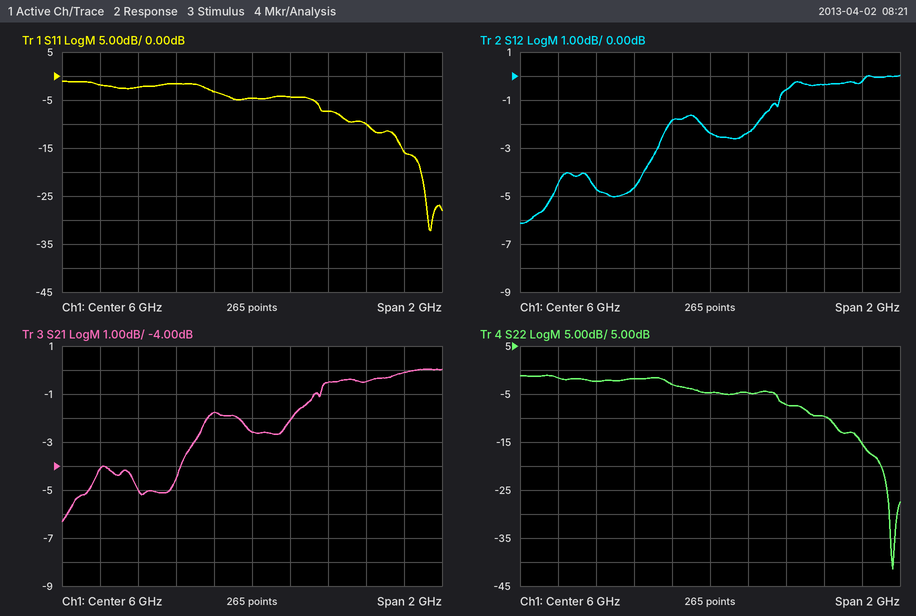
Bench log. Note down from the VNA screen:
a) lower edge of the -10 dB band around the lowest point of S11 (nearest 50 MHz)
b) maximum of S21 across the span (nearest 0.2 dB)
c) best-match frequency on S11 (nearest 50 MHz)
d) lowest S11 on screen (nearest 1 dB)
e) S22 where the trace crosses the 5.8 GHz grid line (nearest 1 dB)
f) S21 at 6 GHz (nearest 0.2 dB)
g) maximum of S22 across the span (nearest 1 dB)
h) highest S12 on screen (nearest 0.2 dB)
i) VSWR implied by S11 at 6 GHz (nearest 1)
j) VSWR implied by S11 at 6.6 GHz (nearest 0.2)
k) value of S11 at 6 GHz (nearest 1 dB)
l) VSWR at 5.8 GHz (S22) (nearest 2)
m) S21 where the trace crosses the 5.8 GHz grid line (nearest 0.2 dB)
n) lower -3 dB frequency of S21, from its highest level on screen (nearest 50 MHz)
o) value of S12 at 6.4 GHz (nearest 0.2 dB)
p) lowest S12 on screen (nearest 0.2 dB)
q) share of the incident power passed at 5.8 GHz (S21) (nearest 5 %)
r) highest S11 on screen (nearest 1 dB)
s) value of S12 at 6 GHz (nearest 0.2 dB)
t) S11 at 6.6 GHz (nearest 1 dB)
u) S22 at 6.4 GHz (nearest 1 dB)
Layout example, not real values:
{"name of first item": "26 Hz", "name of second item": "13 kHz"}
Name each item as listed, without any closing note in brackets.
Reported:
{"lower edge of the -10 dB band around the lowest point of S11": "6.60 GHz", "maximum of S21 across the span": "0.0 dB", "best-match frequency on S11": "6.95 GHz", "lowest S11 on screen": "-32 dB", "S22 where the trace crosses the 5.8 GHz grid line": "-3 dB", "S21 at 6 GHz": "-2.6 dB", "maximum of S22 across the span": "-1 dB", "highest S12 on screen": "0.0 dB", "VSWR implied by S11 at 6 GHz": "4", "VSWR implied by S11 at 6.6 GHz": "2.0", "value of S11 at 6 GHz": "-5 dB", "VSWR at 5.8 GHz (S22)": "6", "S21 where the trace crosses the 5.8 GHz grid line": "-1.8 dB", "lower -3 dB frequency of S21, from its highest level on screen": "5.70 GHz", "value of S12 at 6.4 GHz": "-0.6 dB", "lowest S12 on screen": "-6.2 dB", "share of the incident power passed at 5.8 GHz (S21)": "65 %", "highest S11 on screen": "-1 dB", "value of S12 at 6 GHz": "-2.4 dB", "S11 at 6.6 GHz": "-10 dB", "S22 at 6.4 GHz": "-7 dB"}
